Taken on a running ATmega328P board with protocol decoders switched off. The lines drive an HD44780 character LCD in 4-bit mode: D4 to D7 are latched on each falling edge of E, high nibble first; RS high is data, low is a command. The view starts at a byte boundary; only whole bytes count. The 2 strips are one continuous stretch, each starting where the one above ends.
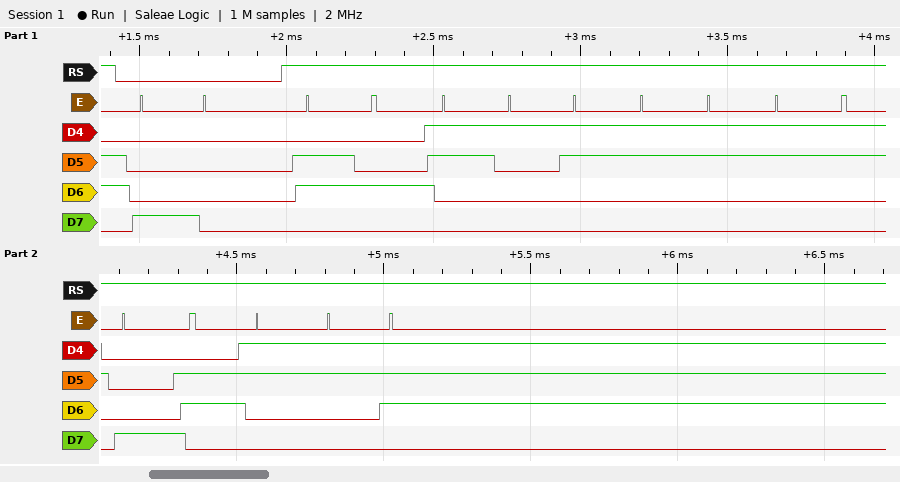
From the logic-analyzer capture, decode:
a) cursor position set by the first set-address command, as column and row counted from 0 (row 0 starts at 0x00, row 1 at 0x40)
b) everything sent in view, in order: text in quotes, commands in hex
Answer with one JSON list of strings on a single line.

["column 0, row 0", "0x80 \"d1338c7\""]
